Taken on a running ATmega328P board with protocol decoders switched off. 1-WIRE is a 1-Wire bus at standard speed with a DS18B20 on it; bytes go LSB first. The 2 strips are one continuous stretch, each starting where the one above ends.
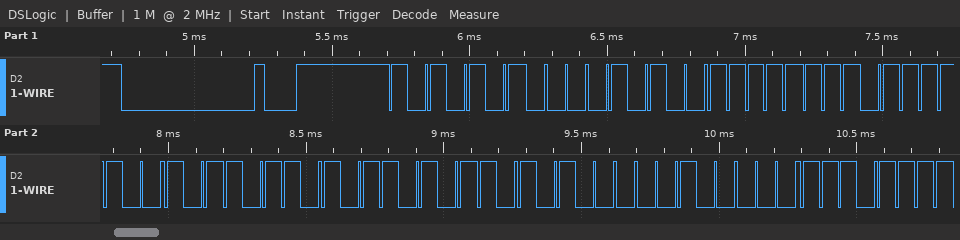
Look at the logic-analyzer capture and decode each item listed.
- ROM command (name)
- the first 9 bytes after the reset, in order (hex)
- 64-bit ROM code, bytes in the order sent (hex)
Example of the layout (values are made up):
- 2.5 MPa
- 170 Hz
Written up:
- Match ROM
- 55 28 FF 3E 6D AD 15 04 F7
- 28 FF 3E 6D AD 15 04 F7
